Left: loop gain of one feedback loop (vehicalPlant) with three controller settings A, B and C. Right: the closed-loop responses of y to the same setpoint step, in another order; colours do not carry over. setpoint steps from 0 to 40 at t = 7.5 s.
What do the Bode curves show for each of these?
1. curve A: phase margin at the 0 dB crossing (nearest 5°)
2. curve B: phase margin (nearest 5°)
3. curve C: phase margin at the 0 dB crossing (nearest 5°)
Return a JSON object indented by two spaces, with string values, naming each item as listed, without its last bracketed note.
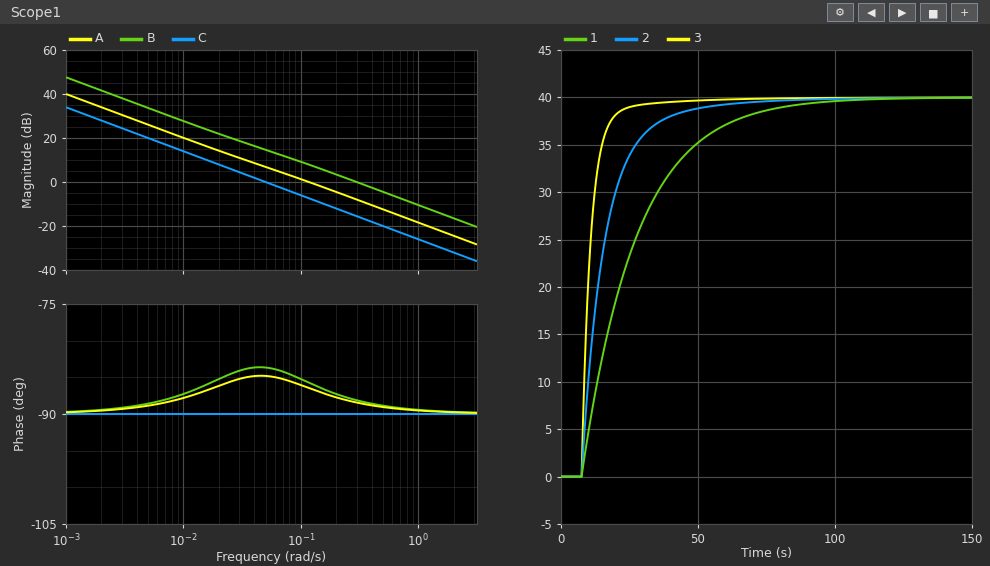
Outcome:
{
  "curve A: phase margin at the 0 dB crossing": "95°",
  "curve B: phase margin": "90°",
  "curve C: phase margin at the 0 dB crossing": "90°"
}
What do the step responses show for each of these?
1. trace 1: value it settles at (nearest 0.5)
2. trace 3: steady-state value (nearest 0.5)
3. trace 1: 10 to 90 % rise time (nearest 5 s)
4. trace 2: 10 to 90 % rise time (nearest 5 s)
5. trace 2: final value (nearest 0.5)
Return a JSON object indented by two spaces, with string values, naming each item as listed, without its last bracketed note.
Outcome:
{
  "trace 1: value it settles at": "40.0",
  "trace 3: steady-state value": "40.0",
  "trace 1: 10 to 90 % rise time": "45 s",
  "trace 2: 10 to 90 % rise time": "20 s",
  "trace 2: final value": "40.0"
}
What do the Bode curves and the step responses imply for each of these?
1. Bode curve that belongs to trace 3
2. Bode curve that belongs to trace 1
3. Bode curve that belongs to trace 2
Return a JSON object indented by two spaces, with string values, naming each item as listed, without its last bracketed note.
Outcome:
{
  "Bode curve that belongs to trace 3": "B",
  "Bode curve that belongs to trace 1": "C",
  "Bode curve that belongs to trace 2": "A"
}
